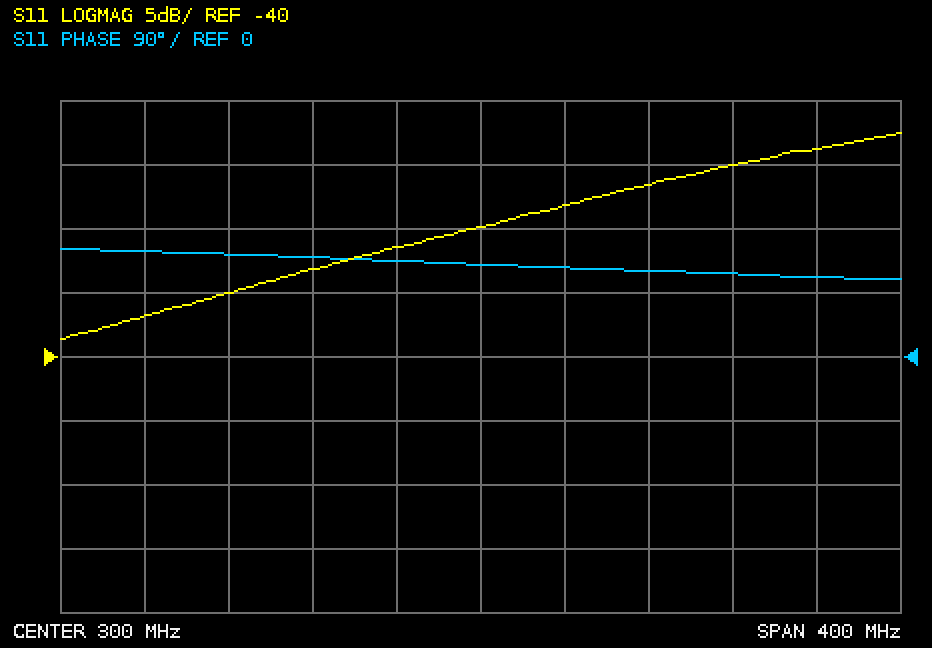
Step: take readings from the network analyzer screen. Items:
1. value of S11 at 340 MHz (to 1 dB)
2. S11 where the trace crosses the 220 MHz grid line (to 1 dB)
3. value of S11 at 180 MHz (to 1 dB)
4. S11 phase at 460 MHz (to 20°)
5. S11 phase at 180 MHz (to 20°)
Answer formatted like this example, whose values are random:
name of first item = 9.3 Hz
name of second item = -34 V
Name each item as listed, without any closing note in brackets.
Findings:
value of S11 at 340 MHz = -28 dB
S11 where the trace crosses the 220 MHz grid line = -33 dB
value of S11 at 180 MHz = -35 dB
S11 phase at 460 MHz = 120°
S11 phase at 180 MHz = 140°
